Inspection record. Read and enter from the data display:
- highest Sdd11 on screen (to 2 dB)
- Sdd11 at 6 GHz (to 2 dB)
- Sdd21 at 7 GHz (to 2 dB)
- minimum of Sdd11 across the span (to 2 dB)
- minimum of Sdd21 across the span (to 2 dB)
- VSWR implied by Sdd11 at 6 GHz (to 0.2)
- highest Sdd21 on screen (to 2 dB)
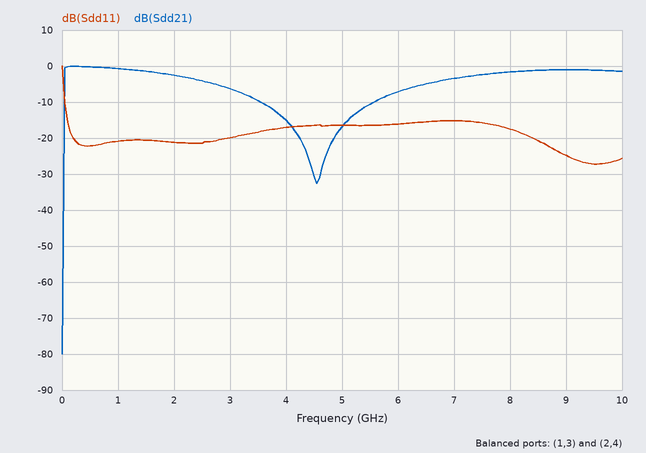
0 dB
-16 dB
-4 dB
-28 dB
-80 dB
1.4
0 dB
